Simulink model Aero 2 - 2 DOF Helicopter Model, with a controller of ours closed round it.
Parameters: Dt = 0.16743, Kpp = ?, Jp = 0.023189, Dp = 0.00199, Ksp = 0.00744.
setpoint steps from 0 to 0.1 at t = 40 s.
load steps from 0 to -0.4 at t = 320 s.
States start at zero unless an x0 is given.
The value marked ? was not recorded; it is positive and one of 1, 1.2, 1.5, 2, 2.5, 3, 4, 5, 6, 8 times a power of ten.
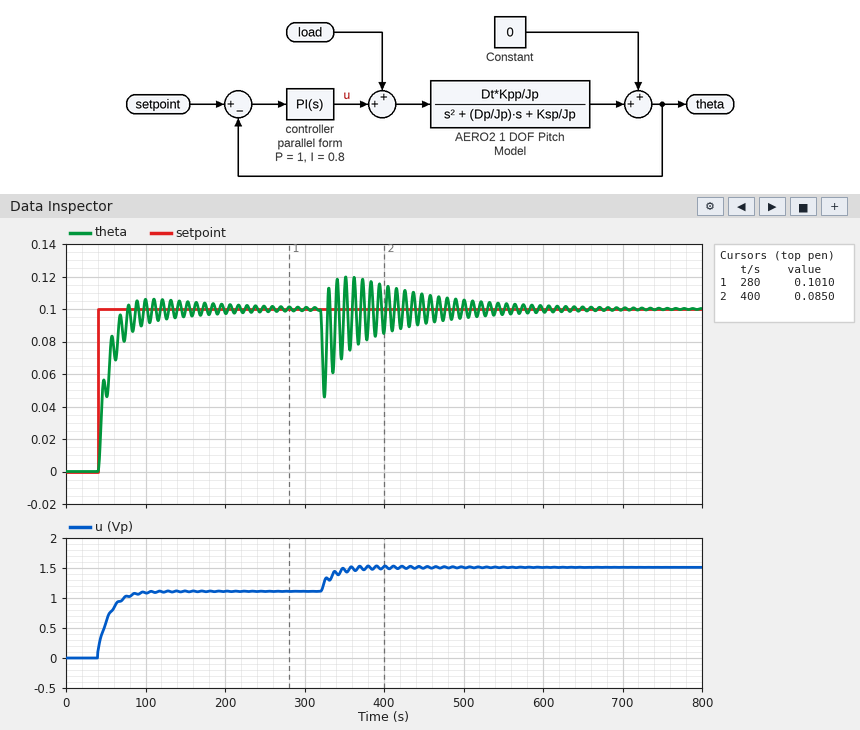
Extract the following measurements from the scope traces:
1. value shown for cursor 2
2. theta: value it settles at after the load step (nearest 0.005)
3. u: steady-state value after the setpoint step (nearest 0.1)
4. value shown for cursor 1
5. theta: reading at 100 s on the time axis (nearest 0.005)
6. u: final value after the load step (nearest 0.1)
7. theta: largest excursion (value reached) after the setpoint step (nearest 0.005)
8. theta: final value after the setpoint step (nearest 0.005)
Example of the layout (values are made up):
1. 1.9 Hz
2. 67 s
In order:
1. 0.0850
2. 0.100
3. 1.1
4. 0.1010
5. 0.105
6. 1.5
7. 0.105
8. 0.100
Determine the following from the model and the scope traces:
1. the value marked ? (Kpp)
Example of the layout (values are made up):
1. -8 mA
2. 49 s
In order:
1. 0.004
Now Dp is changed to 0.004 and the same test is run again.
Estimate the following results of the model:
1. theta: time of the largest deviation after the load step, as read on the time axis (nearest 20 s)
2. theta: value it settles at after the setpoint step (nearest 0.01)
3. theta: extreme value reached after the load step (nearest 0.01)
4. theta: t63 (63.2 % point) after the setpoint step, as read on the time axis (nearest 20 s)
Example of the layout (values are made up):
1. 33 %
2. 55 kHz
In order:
1. 320 s
2. 0.10
3. 0.05
4. 60 s
